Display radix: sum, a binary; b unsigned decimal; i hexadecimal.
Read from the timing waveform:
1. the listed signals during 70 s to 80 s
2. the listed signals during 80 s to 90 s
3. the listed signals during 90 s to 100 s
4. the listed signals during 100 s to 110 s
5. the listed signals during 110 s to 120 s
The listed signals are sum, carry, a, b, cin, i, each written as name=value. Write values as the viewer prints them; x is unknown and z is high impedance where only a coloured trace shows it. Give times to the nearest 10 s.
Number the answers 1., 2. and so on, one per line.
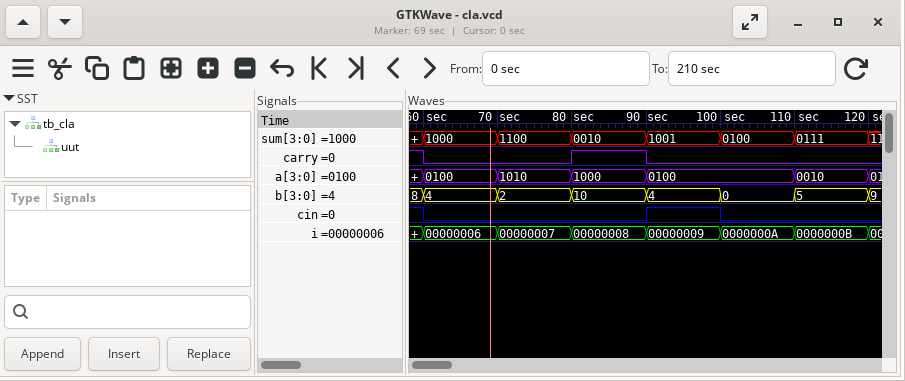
1. sum=1100, carry=0, a=1010, b=2, cin=0, i=00000007
2. sum=0010, carry=1, a=1000, b=10, cin=0, i=00000008
3. sum=1001, carry=0, a=0100, b=4, cin=1, i=00000009
4. sum=0100, carry=0, a=0100, b=0, cin=0, i=0000000A
5. sum=0111, carry=0, a=0010, b=5, cin=0, i=0000000B
